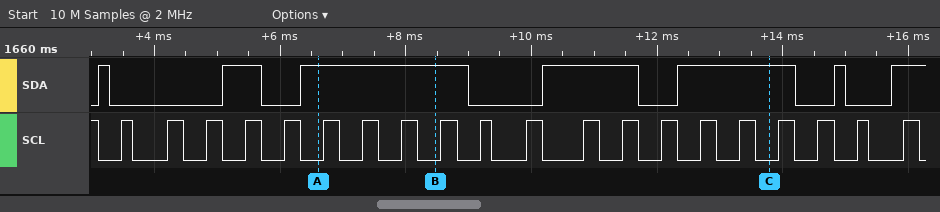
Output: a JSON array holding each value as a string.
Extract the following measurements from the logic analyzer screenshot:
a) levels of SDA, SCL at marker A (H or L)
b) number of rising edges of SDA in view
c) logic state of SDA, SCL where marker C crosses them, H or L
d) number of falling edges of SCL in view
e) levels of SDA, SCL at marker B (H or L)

["SDA=H, SCL=L", "7", "SDA=H, SCL=L", "21", "SDA=H, SCL=L"]
